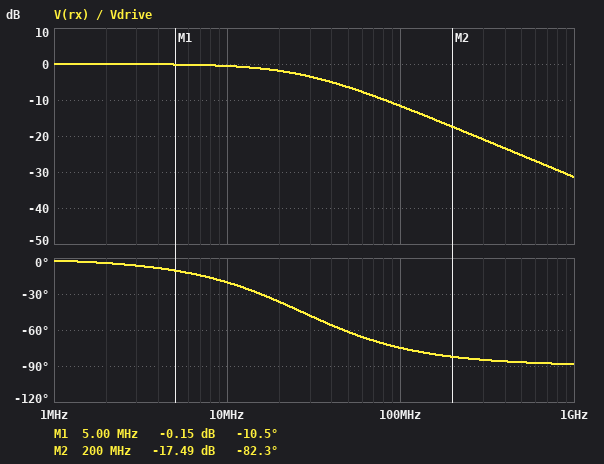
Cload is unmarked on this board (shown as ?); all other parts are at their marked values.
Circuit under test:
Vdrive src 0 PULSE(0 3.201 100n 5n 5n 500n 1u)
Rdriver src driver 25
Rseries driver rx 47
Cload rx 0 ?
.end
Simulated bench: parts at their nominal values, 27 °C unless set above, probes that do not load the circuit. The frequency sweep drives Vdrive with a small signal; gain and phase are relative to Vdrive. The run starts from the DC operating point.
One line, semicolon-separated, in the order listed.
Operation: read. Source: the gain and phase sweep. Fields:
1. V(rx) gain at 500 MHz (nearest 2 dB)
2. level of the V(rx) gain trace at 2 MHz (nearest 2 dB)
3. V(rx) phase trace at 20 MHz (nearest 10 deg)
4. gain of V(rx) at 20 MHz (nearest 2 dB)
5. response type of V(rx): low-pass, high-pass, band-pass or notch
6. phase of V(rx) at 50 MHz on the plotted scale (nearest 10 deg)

-26 dB; 0 dB; -40 deg; -2 dB; low-pass; -60 deg
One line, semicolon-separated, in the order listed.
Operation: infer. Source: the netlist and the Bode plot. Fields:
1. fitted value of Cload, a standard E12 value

82 pF
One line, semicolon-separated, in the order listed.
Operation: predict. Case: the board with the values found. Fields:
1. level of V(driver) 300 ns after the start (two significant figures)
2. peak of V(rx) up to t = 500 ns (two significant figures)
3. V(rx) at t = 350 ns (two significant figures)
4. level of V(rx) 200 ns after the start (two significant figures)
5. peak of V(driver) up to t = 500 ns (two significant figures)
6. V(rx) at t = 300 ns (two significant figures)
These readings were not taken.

3.2 V; 3.2 V; 3.2 V; 3.2 V; 3.2 V; 3.2 V
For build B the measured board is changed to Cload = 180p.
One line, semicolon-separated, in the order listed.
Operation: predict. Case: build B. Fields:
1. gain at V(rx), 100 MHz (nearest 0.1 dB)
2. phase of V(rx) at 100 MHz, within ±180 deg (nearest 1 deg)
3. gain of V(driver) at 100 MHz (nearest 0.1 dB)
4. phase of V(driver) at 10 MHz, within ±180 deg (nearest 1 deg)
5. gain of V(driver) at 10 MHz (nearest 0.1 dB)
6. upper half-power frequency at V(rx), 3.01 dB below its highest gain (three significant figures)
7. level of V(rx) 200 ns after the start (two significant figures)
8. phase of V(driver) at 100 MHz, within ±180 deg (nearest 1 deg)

-18.3 dB; -83 deg; -3.6 dB; -11 deg; -1.1 dB; 12.3 MHz; 3.2 V; -4 deg
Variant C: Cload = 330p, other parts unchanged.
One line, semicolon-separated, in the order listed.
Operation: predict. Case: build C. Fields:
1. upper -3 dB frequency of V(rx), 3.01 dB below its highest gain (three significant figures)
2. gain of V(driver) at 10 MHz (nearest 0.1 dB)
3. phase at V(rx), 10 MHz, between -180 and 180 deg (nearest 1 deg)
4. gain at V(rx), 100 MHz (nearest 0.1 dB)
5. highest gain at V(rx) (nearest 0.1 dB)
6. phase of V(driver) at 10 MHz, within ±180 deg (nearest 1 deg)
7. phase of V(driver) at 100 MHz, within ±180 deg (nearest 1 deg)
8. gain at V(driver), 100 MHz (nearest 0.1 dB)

6.70 MHz; -2.2 dB; -56 deg; -23.5 dB; 0 dB; -12 deg; -2 deg; -3.7 dB
